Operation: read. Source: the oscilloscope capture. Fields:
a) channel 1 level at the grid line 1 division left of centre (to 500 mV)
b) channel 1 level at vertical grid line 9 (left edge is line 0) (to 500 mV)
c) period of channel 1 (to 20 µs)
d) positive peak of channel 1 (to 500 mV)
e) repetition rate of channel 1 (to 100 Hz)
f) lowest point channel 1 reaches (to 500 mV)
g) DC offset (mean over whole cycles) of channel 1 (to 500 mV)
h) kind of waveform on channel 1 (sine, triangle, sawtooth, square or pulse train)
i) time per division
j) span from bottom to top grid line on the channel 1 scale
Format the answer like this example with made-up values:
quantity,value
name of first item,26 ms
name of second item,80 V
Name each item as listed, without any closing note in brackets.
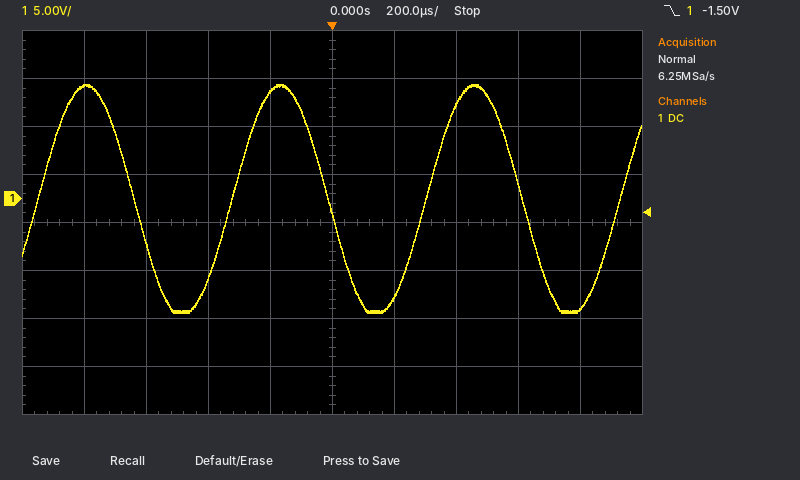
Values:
quantity,value
channel 1 level at the grid line 1 division left of centre,11.0 V
channel 1 level at vertical grid line 9 (left edge is line 0),-11.5 V
period of channel 1,620 µs
positive peak of channel 1,12.0 V
repetition rate of channel 1,1.6 kHz
lowest point channel 1 reaches,-12.0 V
DC offset (mean over whole cycles) of channel 1,0.0 V
kind of waveform on channel 1,sine
time per division,200 µs
span from bottom to top grid line on the channel 1 scale,40 V
